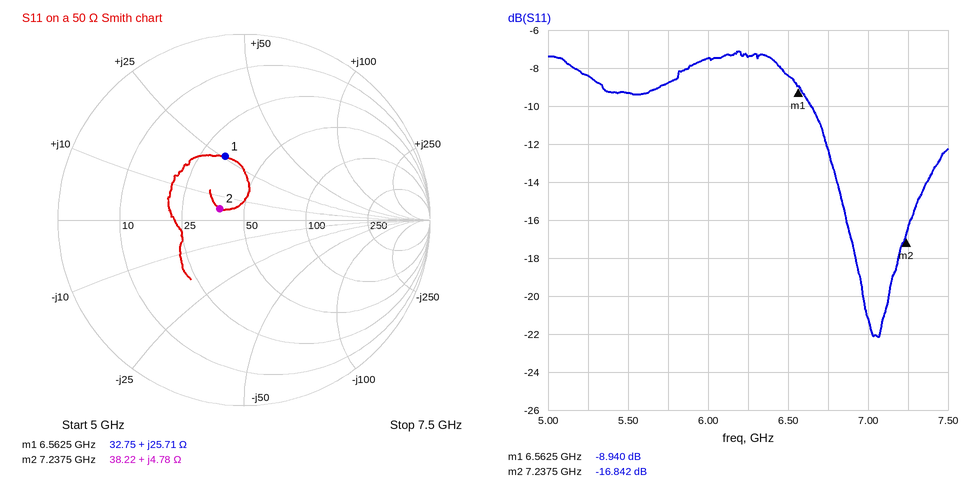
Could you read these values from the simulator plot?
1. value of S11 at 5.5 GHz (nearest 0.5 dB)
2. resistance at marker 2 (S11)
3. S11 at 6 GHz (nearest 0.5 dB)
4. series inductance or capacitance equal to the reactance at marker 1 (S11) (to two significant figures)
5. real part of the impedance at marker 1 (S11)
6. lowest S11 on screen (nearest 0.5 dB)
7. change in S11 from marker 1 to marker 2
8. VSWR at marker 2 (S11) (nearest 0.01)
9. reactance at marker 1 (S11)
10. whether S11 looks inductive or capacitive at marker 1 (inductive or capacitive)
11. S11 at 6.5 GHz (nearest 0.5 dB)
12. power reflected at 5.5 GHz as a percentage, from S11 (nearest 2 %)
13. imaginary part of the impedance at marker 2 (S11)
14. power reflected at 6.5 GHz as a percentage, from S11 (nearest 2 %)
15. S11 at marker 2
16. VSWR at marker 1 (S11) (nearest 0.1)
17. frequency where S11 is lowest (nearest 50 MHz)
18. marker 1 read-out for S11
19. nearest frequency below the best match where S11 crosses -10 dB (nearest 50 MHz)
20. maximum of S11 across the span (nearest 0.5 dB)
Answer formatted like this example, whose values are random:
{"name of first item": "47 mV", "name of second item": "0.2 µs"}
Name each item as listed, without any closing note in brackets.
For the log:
{"value of S11 at 5.5 GHz": "-9.5 dB", "resistance at marker 2": "38.22 Ω", "S11 at 6 GHz": "-7.5 dB", "series inductance or capacitance equal to the reactance at marker 1 (S11)": "620 pH", "real part of the impedance at marker 1": "32.75 Ω", "lowest S11 on screen": "-22.0 dB", "change in S11 from marker 1 to marker 2": "-7.902 dB", "VSWR at marker 2 (S11)": "1.34", "reactance at marker 1": "+25.71 Ω", "whether S11 looks inductive or capacitive at marker 1": "inductive", "S11 at 6.5 GHz": "-8.5 dB", "power reflected at 5.5 GHz as a percentage, from S11": "12 %", "imaginary part of the impedance at marker 2": "+4.78 Ω", "power reflected at 6.5 GHz as a percentage, from S11": "14 %", "S11 at marker 2": "-16.842 dB", "VSWR at marker 1 (S11)": "2.1", "frequency where S11 is lowest": "7.05 GHz", "marker 1 read-out for S11": "-8.940 dB", "nearest frequency below the best match where S11 crosses -10 dB": "6.65 GHz", "maximum of S11 across the span": "-7.0 dB"}
